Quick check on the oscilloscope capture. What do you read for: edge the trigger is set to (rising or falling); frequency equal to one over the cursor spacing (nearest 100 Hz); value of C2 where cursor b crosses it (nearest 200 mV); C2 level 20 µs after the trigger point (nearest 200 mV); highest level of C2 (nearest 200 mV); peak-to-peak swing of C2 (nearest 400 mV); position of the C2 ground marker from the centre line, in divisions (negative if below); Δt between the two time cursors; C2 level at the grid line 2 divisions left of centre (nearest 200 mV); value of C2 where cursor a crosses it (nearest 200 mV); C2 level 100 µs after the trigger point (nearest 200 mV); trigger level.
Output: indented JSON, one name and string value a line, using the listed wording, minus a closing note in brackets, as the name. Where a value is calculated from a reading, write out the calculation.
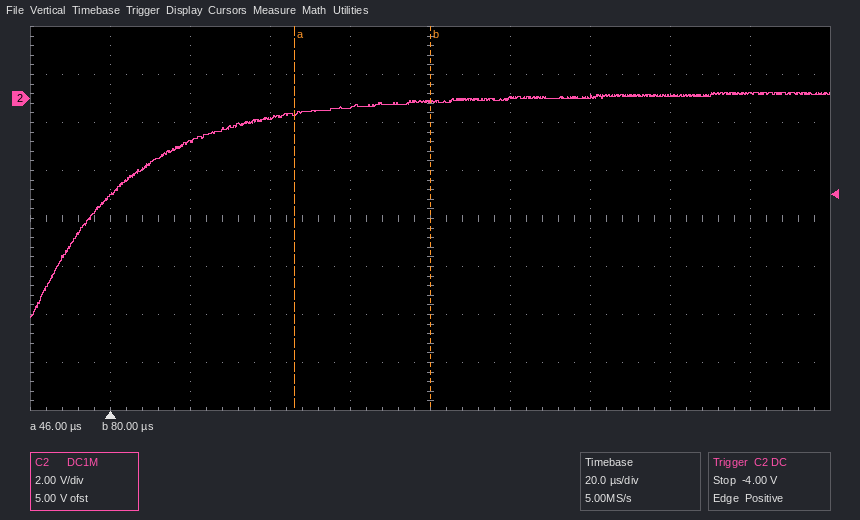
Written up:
{
  "edge the trigger is set to": "rising",
  "frequency equal to one over the cursor spacing": "1 / 34 µs ≈ 29.4 kHz",
  "value of C2 where cursor b crosses it": "-200 mV",
  "C2 level 20 µs after the trigger point": "-1.8 V",
  "highest level of C2": "200 mV",
  "peak-to-peak swing of C2": "9.2 V",
  "position of the C2 ground marker from the centre line, in divisions": "+2.5 div",
  "Δt between the two time cursors": "80 µs − (46 µs) = 34 µs",
  "C2 level at the grid line 2 divisions left of centre": "-800 mV",
  "value of C2 where cursor a crosses it": "-600 mV",
  "C2 level 100 µs after the trigger point": "0.0 V",
  "trigger level": "-4.00 V"
}
